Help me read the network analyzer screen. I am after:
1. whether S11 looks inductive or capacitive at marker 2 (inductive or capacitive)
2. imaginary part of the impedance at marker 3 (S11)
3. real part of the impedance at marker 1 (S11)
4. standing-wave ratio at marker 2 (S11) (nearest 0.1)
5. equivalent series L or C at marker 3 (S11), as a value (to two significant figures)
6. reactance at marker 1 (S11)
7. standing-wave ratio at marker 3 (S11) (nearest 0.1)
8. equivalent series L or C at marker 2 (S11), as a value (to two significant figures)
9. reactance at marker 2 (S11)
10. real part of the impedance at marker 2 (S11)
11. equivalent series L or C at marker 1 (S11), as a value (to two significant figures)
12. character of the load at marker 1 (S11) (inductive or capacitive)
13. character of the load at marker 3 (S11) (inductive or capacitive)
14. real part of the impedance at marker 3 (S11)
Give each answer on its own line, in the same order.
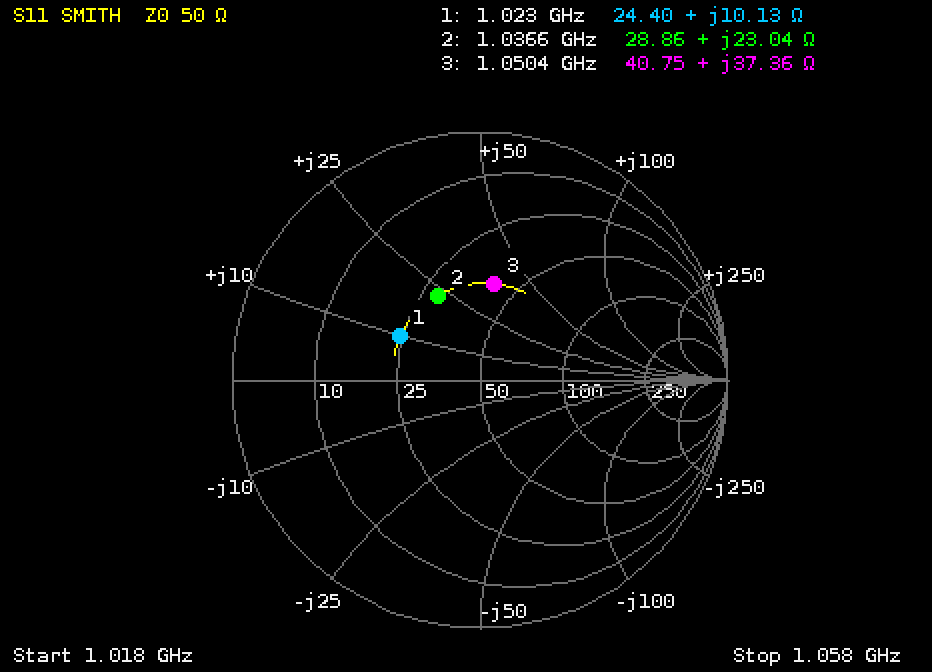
inductive
+37.36 Ω
24.40 Ω
2.2
5.7 nH
+10.13 Ω
2.3
3.5 nH
+23.04 Ω
28.86 Ω
1.6 nH
inductive
inductive
40.75 Ω
